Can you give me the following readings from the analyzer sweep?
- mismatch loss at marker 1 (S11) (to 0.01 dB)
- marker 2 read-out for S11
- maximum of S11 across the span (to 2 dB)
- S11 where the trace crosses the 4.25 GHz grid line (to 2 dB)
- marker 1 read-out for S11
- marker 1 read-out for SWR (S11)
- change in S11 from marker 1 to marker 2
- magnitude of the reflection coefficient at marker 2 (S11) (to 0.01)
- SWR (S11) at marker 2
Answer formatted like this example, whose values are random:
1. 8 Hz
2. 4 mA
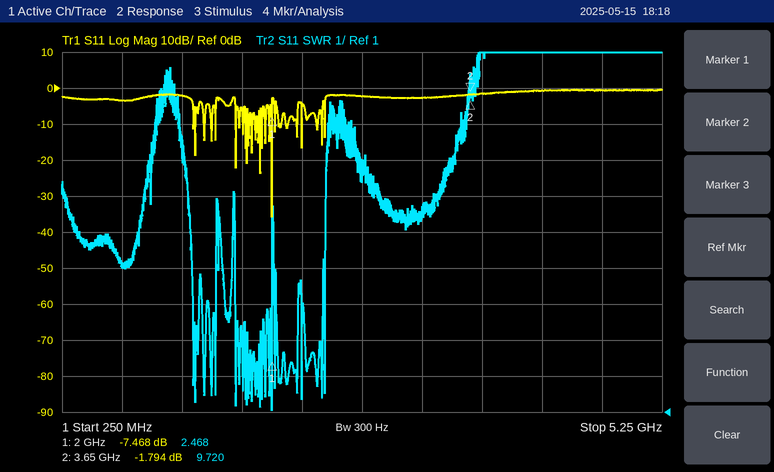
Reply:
1. 0.86 dB
2. -1.794 dB
3. 0 dB
4. 0 dB
5. -7.468 dB
6. 2.468
7. 5.674 dB
8. 0.81
9. 9.720
